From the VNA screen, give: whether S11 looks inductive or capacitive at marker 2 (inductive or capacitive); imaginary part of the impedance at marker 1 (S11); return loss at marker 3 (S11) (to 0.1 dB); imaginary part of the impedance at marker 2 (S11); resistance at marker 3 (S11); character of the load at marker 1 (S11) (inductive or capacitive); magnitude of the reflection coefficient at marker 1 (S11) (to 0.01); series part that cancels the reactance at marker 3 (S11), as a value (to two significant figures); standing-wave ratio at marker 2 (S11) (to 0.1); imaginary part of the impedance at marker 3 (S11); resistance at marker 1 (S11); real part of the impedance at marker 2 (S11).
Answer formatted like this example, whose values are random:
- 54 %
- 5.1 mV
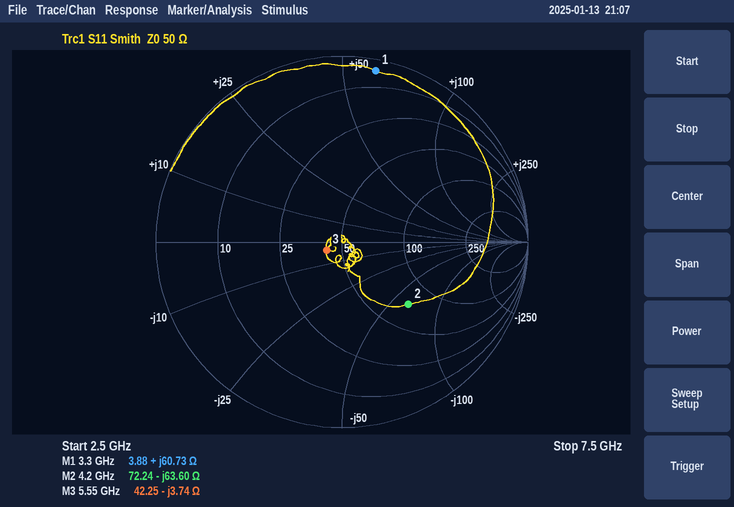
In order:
- capacitive
- +60.73 Ω
- 20.6 dB
- -63.60 Ω
- 42.25 Ω
- inductive
- 0.94
- 110 pH
- 2.9
- -3.74 Ω
- 3.88 Ω
- 72.24 Ω
